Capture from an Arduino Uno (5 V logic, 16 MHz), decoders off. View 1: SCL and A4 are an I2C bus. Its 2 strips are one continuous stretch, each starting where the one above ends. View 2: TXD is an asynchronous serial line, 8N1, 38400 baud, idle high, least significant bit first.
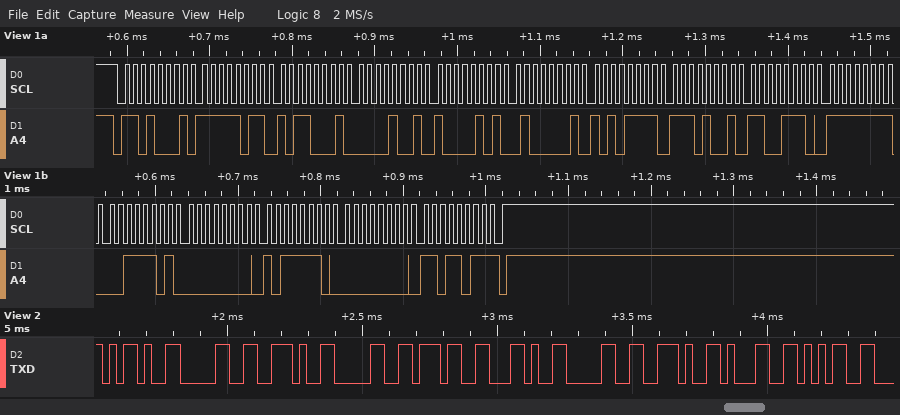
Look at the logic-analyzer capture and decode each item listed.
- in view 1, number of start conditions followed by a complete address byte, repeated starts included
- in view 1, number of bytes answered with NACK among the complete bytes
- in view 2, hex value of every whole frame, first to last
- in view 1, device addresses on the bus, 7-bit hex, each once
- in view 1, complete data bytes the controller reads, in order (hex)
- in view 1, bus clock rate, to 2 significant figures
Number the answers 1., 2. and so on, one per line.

1. 1
2. 1
3. 0x2D 0x30 0x2E 0x30 0x37 0x2C 0x30 0x2E 0x31 0x35
4. 0x68
5. FB B1 09 85 41 AF E9 CE FF 3D 00 BE 00 DB
6. 100 kHz
